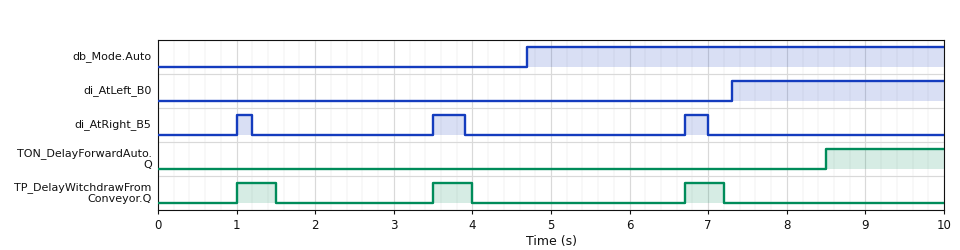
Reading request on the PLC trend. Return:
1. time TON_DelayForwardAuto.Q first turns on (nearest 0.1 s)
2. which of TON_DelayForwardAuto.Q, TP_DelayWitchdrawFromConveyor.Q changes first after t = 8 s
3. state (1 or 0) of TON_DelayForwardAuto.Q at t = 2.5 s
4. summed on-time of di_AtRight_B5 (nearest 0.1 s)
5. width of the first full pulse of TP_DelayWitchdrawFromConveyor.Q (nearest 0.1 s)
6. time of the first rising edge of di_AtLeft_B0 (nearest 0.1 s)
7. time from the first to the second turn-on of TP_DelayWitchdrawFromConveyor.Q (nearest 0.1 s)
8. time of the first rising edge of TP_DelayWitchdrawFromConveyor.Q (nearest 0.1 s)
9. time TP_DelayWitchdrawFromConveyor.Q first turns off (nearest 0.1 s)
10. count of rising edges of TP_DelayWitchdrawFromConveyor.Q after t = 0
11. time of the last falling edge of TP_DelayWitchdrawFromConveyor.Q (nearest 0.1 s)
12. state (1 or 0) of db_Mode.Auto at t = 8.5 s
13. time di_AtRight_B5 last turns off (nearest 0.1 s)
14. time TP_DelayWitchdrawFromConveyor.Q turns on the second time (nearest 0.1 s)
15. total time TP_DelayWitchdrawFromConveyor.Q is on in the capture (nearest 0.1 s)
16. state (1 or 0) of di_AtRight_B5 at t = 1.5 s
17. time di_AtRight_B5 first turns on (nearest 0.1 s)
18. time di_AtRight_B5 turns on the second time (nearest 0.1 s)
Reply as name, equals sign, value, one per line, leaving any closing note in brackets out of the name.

time TON_DelayForwardAuto.Q first turns on = 8.5 s
which of TON_DelayForwardAuto.Q, TP_DelayWitchdrawFromConveyor.Q changes first after t = 8 s = TON_DelayForwardAuto.Q
state (1 or 0) of TON_DelayForwardAuto.Q at t = 2.5 s = 0
summed on-time of di_AtRight_B5 = 0.9 s
width of the first full pulse of TP_DelayWitchdrawFromConveyor.Q = 0.5 s
time of the first rising edge of di_AtLeft_B0 = 7.3 s
time from the first to the second turn-on of TP_DelayWitchdrawFromConveyor.Q = 2.5 s
time of the first rising edge of TP_DelayWitchdrawFromConveyor.Q = 1.0 s
time TP_DelayWitchdrawFromConveyor.Q first turns off = 1.5 s
count of rising edges of TP_DelayWitchdrawFromConveyor.Q after t = 0 = 3
time of the last falling edge of TP_DelayWitchdrawFromConveyor.Q = 7.2 s
state (1 or 0) of db_Mode.Auto at t = 8.5 s = 1
time di_AtRight_B5 last turns off = 7.0 s
time TP_DelayWitchdrawFromConveyor.Q turns on the second time = 3.5 s
total time TP_DelayWitchdrawFromConveyor.Q is on in the capture = 1.5 s
state (1 or 0) of di_AtRight_B5 at t = 1.5 s = 0
time di_AtRight_B5 first turns on = 1.0 s
time di_AtRight_B5 turns on the second time = 3.5 s
